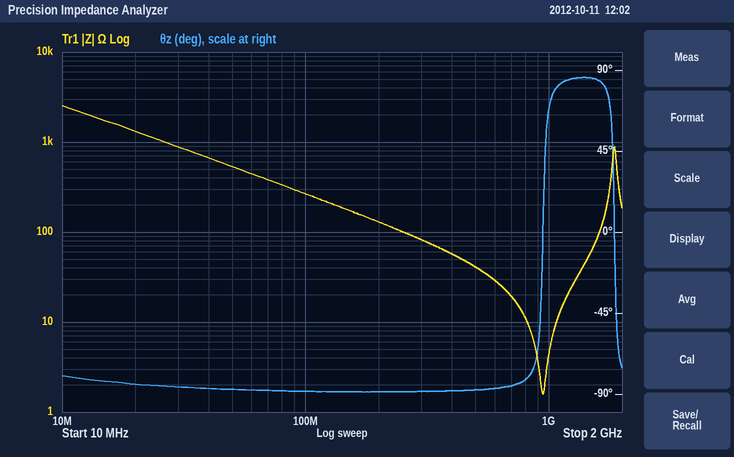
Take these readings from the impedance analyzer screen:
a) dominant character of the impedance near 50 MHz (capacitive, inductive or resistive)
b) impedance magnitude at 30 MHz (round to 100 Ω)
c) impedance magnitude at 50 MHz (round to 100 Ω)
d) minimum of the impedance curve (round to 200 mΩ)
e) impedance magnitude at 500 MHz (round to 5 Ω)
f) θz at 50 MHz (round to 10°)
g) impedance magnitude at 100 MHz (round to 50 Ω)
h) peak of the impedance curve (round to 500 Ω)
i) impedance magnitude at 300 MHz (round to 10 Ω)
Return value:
capacitive
900 Ω
500 Ω
1.6 Ω
40 Ω
-90°
250 Ω
2.5 kΩ
80 Ω
